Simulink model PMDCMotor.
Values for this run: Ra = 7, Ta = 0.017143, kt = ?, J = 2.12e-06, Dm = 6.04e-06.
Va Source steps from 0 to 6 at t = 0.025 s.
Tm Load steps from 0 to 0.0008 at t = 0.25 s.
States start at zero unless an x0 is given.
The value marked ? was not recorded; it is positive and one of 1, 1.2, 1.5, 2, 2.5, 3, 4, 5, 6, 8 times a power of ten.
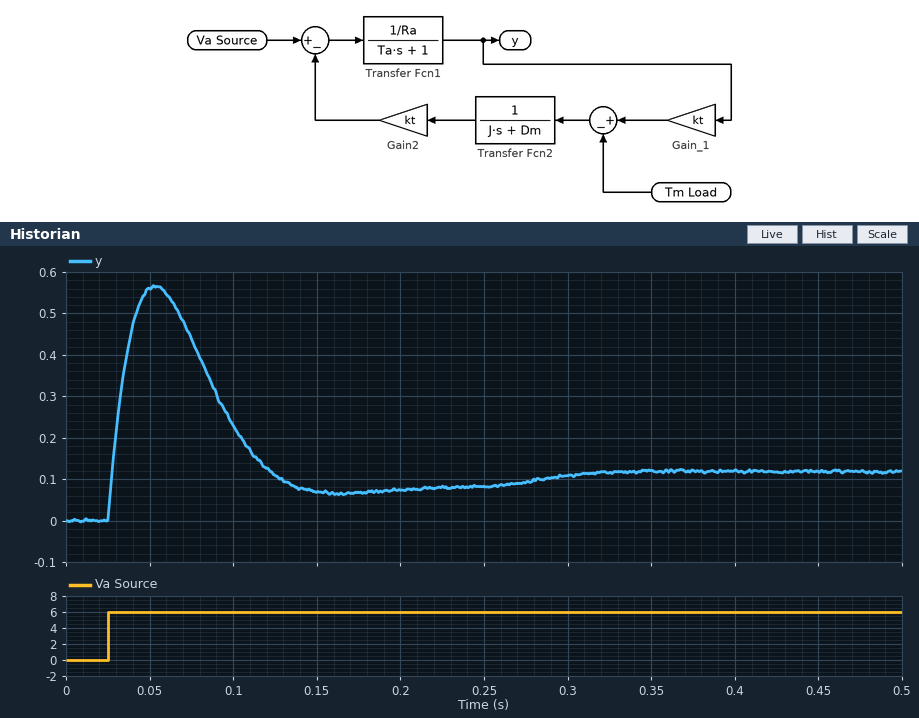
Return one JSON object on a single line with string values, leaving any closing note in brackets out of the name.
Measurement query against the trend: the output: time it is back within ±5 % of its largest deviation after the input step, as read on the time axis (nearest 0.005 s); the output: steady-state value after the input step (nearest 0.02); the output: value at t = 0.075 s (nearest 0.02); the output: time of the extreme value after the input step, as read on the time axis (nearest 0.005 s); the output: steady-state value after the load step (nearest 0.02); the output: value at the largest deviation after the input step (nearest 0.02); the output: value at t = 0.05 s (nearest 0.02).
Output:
{"the output: time it is back within ±5 % of its largest deviation after the input step, as read on the time axis": "0.125 s", "the output: steady-state value after the input step": "0.08", "the output: value at t = 0.075 s": "0.44", "the output: time of the extreme value after the input step, as read on the time axis": "0.055 s", "the output: steady-state value after the load step": "0.12", "the output: value at the largest deviation after the input step": "0.56", "the output: value at t = 0.05 s": "0.56"}
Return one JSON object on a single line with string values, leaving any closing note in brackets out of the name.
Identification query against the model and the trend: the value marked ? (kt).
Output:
{"the value marked ?": "0.02"}
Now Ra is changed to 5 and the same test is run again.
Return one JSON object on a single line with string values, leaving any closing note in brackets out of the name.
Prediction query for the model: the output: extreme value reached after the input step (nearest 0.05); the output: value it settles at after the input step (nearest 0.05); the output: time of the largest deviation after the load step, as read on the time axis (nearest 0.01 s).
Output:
{"the output: extreme value reached after the input step": "0.75", "the output: value it settles at after the input step": "0.10", "the output: time of the largest deviation after the load step, as read on the time axis": "0.33 s"}
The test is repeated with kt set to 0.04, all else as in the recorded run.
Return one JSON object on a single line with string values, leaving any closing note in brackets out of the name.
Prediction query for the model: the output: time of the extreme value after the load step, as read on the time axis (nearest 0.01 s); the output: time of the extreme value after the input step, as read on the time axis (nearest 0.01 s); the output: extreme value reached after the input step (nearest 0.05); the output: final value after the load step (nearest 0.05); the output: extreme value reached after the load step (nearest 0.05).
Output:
{"the output: time of the extreme value after the load step, as read on the time axis": "0.29 s", "the output: time of the extreme value after the input step, as read on the time axis": "0.04 s", "the output: extreme value reached after the input step": "0.40", "the output: final value after the load step": "0.05", "the output: extreme value reached after the load step": "0.05"}
